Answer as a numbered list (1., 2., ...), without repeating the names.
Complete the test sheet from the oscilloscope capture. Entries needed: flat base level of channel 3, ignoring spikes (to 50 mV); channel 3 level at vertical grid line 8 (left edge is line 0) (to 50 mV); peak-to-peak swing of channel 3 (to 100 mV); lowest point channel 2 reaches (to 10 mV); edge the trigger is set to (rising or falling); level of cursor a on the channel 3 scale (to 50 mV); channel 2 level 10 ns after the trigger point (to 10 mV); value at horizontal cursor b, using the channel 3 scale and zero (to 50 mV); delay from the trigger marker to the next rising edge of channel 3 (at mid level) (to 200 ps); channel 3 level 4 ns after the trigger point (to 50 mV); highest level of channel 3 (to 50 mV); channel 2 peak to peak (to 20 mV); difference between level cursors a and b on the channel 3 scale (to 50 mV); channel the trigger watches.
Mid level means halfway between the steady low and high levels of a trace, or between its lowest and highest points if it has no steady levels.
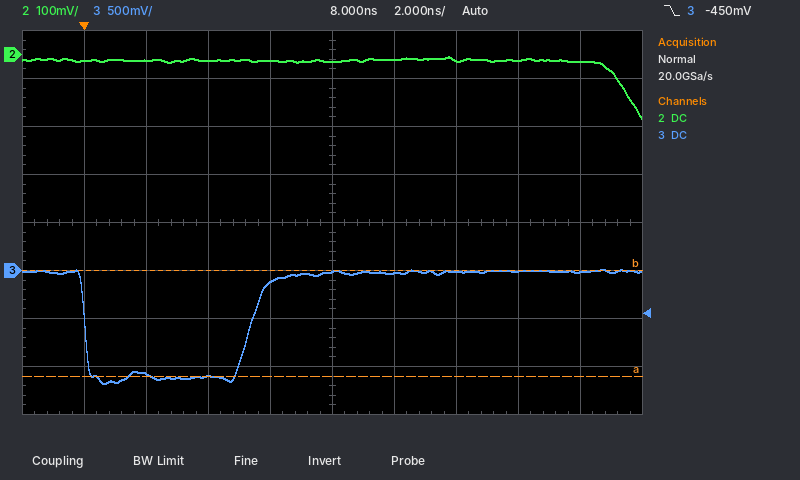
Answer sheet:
1. -1.10 V
2. 0 mV
3. 1.20 V
4. -130 mV
5. falling
6. -1.10 V
7. -10 mV
8. 0 mV
9. 5.4 ns
10. -1.10 V
11. 0 mV
12. 120 mV
13. 1.10 V
14. channel 3
